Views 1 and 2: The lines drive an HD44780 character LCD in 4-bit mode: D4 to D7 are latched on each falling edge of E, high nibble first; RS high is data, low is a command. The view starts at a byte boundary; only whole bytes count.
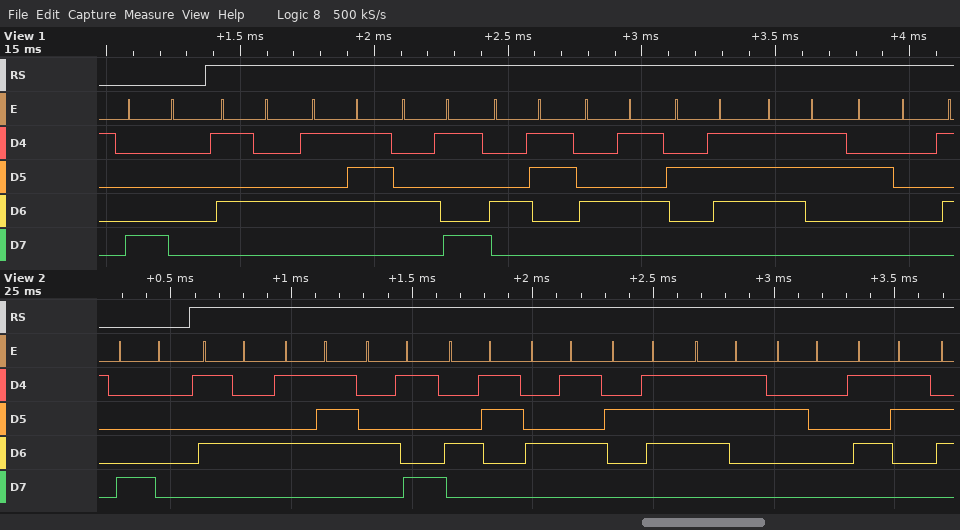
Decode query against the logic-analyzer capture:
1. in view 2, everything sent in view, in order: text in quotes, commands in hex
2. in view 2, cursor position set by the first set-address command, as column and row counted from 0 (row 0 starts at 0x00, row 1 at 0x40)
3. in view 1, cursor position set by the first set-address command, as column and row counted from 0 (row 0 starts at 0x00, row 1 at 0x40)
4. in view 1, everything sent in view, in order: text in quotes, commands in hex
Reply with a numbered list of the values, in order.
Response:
1. 0x80 "TWICE's S"
2. column 0, row 0
3. column 0, row 0
4. 0x80 "TWICE's "
